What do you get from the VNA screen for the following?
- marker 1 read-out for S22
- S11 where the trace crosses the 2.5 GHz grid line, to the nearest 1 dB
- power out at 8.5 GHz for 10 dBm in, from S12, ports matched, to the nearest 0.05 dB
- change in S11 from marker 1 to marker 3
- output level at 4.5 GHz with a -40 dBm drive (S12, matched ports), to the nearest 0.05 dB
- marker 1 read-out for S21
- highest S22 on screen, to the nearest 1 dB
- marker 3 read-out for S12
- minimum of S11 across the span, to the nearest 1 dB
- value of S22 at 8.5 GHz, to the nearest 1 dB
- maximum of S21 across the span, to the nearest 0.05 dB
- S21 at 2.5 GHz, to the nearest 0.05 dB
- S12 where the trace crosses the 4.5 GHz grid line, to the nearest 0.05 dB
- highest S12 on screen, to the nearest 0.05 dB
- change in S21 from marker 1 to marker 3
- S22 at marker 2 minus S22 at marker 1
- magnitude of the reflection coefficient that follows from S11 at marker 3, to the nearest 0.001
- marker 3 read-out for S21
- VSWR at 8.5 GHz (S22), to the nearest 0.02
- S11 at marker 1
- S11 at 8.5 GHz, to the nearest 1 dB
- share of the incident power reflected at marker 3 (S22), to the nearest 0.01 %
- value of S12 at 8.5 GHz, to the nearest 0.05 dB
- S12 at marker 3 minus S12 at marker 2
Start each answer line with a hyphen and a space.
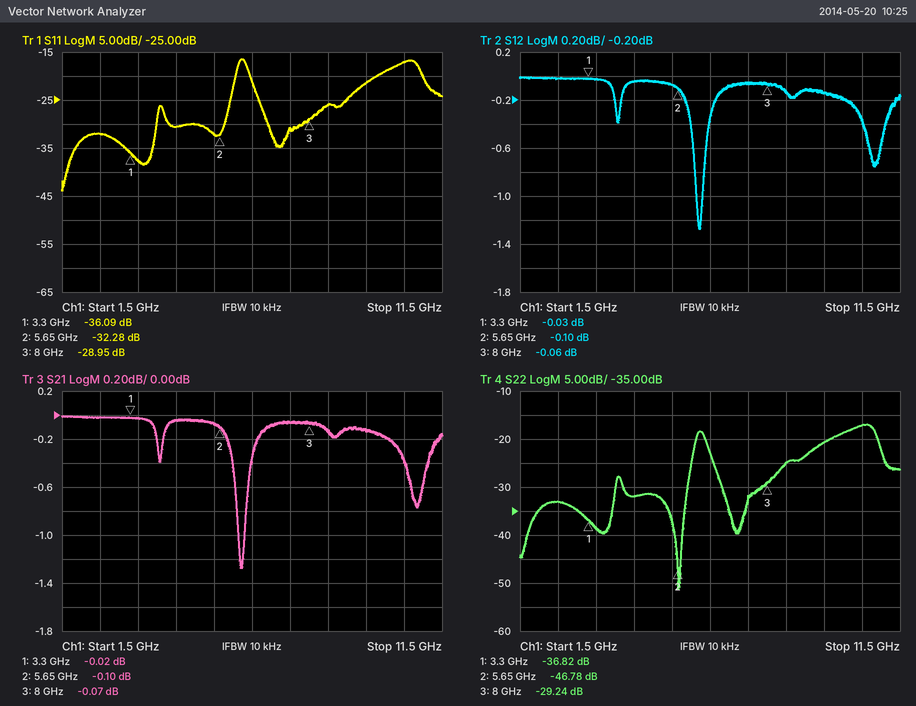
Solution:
- -36.82 dB
- -32 dB
- 9.85 dBm
- 7.14 dB
- -40.05 dBm
- -0.02 dB
- -17 dB
- -0.06 dB
- -44 dB
- -25 dB
- 0.00 dB
- 0.00 dB
- -0.05 dB
- 0.00 dB
- -0.05 dB
- -9.96 dB
- 0.036
- -0.07 dB
- 1.12
- -36.09 dB
- -26 dB
- 0.12 %
- -0.15 dB
- 0.04 dB
